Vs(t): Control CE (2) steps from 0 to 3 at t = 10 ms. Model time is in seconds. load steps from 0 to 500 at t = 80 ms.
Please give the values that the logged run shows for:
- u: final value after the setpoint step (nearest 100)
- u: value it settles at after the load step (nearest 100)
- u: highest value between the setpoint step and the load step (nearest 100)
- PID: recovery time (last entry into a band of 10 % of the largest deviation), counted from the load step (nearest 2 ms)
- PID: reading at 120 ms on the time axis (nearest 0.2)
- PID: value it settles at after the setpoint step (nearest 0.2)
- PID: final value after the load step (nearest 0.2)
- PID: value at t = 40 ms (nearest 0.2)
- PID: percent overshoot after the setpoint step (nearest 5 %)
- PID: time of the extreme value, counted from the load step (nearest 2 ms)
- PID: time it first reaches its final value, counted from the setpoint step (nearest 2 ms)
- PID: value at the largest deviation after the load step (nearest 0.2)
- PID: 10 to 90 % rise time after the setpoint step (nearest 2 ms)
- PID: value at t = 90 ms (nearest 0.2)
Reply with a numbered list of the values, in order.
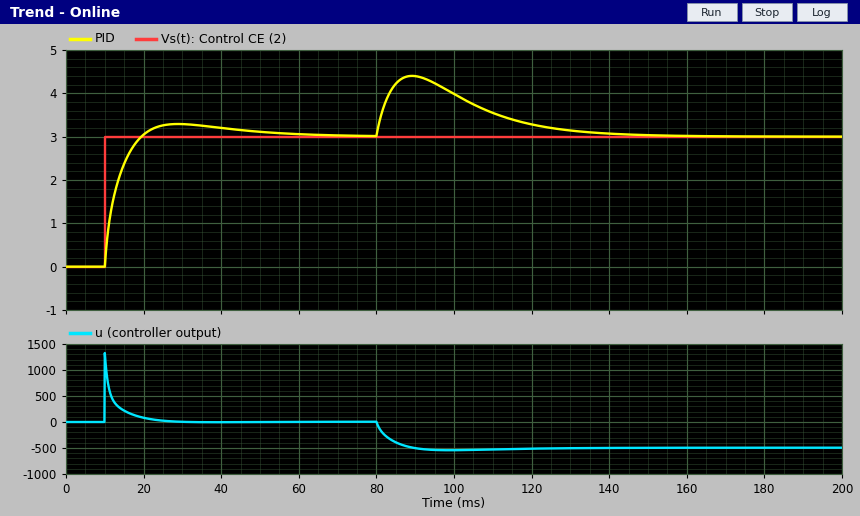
1. 0
2. -500
3. 1300
4. 50 ms
5. 3.2
6. 3.0
7. 3.0
8. 3.2
9. 10 %
10. 10 ms
11. 10 ms
12. 4.4
13. 6 ms
14. 4.4
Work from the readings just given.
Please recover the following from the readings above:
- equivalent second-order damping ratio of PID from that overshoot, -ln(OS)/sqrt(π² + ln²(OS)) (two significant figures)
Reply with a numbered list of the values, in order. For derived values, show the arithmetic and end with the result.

1. ln(0.1) = -2.303; 2.303 / sqrt(9.870 + 5.302) = 0.59
